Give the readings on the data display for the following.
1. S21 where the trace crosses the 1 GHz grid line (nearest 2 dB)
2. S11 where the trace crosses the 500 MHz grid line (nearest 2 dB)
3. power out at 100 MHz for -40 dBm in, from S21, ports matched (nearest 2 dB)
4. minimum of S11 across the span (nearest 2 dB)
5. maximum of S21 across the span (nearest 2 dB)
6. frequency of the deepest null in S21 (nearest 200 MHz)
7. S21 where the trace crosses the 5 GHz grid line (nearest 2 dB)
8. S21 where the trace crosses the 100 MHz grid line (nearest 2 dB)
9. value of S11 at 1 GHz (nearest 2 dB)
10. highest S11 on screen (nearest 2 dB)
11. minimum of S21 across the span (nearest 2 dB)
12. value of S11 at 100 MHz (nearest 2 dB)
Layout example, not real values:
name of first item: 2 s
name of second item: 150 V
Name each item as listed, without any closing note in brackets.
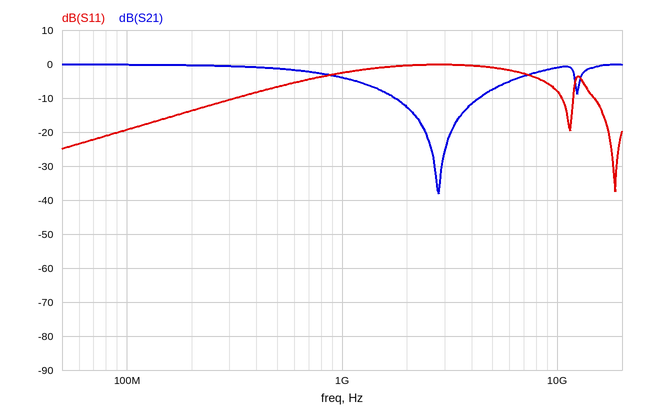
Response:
S21 where the trace crosses the 1 GHz grid line: -4 dB
S11 where the trace crosses the 500 MHz grid line: -6 dB
power out at 100 MHz for -40 dBm in, from S21, ports matched: -40 dBm
minimum of S11 across the span: -38 dB
maximum of S21 across the span: 0 dB
frequency of the deepest null in S21: 2.8 GHz
S21 where the trace crosses the 5 GHz grid line: -8 dB
S21 where the trace crosses the 100 MHz grid line: 0 dB
value of S11 at 1 GHz: -2 dB
highest S11 on screen: 0 dB
minimum of S21 across the span: -38 dB
value of S11 at 100 MHz: -20 dB
